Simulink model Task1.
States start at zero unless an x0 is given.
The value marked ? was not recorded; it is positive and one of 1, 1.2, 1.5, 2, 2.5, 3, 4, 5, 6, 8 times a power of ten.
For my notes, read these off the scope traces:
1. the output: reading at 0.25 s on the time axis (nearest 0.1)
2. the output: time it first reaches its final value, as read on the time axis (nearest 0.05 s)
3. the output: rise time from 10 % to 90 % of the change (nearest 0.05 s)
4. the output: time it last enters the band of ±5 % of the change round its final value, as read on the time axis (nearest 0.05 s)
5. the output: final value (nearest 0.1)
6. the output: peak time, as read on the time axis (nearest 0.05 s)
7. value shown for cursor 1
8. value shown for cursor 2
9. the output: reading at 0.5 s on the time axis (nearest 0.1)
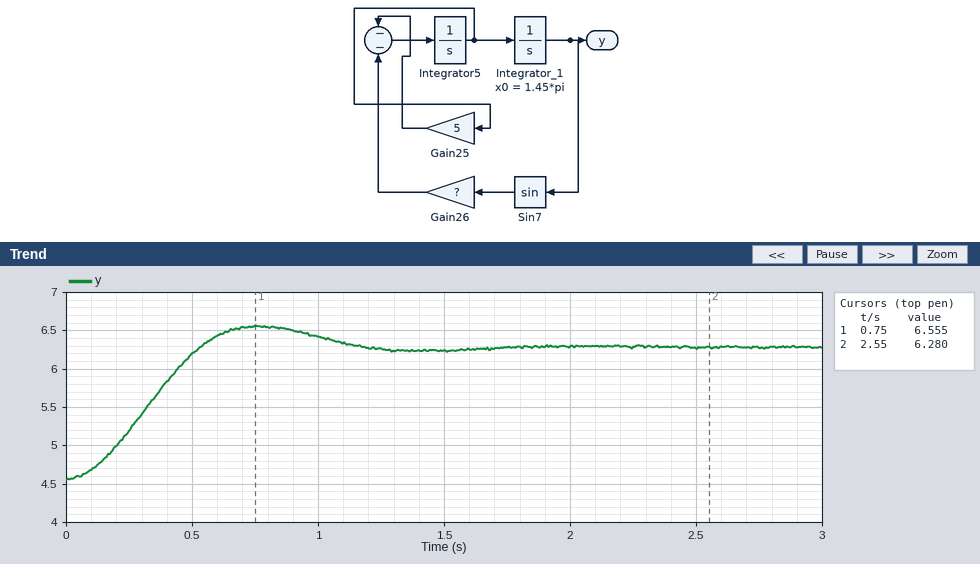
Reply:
5.2
0.55 s
0.35 s
1.05 s
6.3
0.75 s
6.555
6.280
6.2
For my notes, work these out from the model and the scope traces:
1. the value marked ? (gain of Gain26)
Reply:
30
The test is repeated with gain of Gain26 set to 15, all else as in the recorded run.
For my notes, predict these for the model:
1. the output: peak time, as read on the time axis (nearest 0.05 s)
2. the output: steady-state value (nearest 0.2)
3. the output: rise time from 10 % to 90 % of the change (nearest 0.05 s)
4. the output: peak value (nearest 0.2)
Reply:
1.30 s
6.2
0.65 s
6.4
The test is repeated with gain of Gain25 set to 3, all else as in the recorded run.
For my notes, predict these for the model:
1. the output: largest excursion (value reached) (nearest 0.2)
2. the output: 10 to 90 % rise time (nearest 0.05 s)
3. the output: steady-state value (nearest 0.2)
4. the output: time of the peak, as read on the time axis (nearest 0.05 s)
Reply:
6.8
0.30 s
6.2
0.70 s
